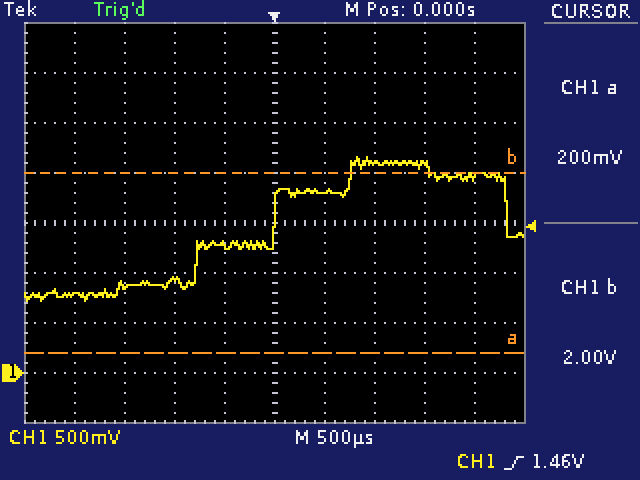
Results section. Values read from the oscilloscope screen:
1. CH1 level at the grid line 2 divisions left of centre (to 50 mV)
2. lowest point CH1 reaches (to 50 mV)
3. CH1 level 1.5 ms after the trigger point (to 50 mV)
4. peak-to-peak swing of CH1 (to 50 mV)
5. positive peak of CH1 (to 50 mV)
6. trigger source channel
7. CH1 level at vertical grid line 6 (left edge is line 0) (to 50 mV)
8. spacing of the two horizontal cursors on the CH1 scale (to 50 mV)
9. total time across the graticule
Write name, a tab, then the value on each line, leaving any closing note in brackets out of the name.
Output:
CH1 level at the grid line 2 divisions left of centre	950 mV
lowest point CH1 reaches	700 mV
CH1 level 1.5 ms after the trigger point	2.10 V
peak-to-peak swing of CH1	1.45 V
positive peak of CH1	2.15 V
trigger source channel	CH1
CH1 level at vertical grid line 6 (left edge is line 0)	1.80 V
spacing of the two horizontal cursors on the CH1 scale	1.80 V
total time across the graticule	5 ms
